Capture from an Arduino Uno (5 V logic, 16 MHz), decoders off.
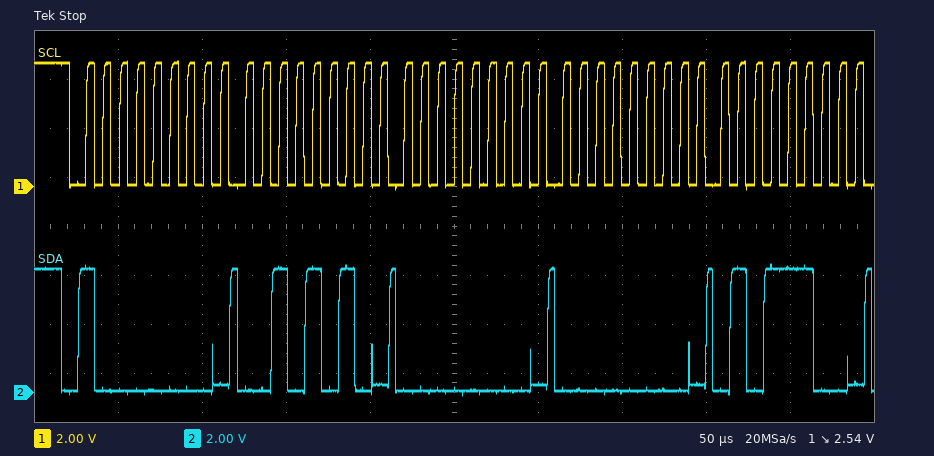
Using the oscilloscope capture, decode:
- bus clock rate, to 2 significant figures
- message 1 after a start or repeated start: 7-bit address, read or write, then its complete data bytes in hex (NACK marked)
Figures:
100 kHz
0x40 write: 2A 00 00 5C
